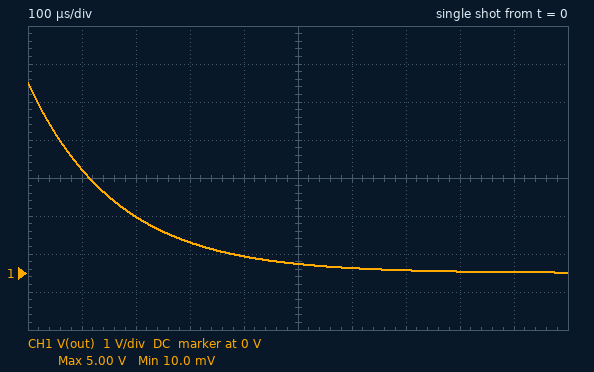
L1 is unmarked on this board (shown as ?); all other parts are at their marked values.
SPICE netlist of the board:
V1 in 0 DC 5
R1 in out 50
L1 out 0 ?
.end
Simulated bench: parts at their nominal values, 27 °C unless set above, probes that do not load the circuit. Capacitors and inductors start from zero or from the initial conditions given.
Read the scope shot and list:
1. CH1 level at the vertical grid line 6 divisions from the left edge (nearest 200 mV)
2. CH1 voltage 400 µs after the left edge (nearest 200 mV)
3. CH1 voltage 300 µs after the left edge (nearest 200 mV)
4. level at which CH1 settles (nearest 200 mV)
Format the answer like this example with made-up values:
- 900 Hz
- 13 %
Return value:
- 200 mV
- 400 mV
- 800 mV
- 0 V
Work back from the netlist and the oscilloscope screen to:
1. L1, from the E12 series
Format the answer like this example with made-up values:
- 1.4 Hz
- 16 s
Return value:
- 8.2 mH
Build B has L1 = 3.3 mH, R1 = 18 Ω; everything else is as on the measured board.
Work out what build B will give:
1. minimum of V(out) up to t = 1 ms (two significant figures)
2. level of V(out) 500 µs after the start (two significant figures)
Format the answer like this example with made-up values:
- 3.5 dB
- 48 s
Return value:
- 21 mV
- 330 mV
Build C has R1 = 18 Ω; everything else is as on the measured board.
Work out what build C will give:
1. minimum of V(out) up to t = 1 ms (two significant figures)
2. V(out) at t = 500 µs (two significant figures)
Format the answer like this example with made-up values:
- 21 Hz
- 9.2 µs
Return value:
- 560 mV
- 1.7 V
